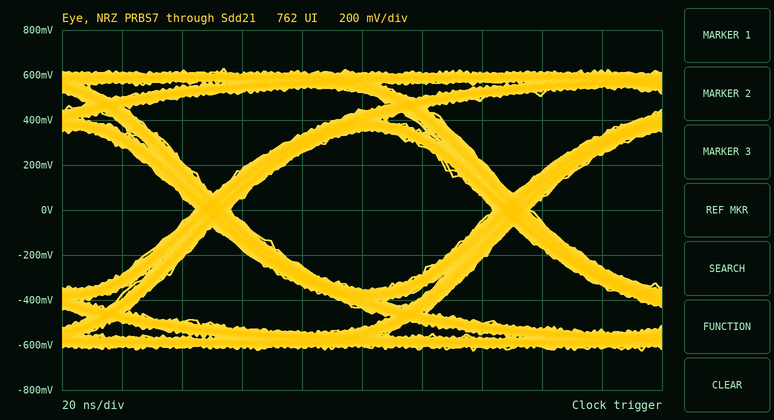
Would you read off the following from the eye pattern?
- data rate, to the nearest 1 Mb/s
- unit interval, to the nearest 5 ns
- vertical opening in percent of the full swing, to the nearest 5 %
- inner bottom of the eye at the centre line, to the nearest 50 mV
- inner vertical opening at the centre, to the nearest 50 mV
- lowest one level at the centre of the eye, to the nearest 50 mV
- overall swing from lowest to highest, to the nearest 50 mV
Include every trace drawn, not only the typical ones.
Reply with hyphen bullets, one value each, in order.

- 10 Mb/s
- 100 ns
- 55 %
- -350 mV
- 700 mV
- 350 mV
- 1.25 V
